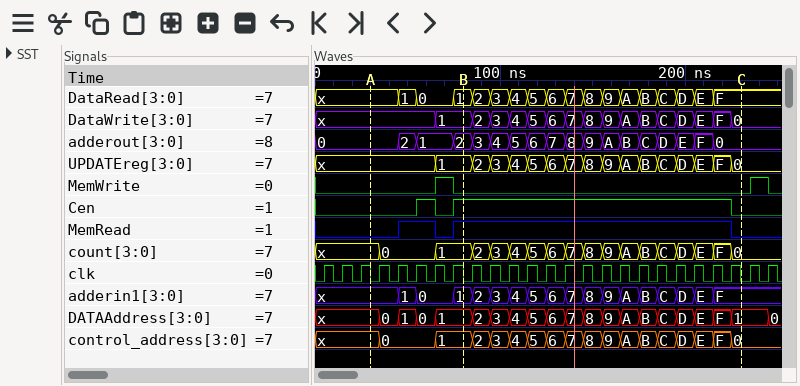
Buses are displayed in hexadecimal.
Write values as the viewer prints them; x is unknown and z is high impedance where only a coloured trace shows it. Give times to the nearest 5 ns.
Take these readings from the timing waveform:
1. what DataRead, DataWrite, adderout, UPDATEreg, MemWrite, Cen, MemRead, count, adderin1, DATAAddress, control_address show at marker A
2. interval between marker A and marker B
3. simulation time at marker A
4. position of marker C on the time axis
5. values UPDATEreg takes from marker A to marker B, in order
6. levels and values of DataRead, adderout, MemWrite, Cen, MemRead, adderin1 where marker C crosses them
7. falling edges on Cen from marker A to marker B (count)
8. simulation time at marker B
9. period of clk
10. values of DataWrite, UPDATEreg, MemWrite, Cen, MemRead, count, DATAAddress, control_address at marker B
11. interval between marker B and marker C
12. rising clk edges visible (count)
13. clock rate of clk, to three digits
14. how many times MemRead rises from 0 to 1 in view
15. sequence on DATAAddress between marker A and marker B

DataRead=x, DataWrite=x, adderout=0, UPDATEreg=x, MemWrite=0, Cen=0, MemRead=0, count=x, adderin1=x, DATAAddress=x, control_address=x
50 ns
30 ns
230 ns
x, 1
DataRead=F, adderout=0, MemWrite=0, Cen=0, MemRead=0, adderin1=F
1
80 ns
10 ns
DataWrite=1, UPDATEreg=1, MemWrite=0, Cen=1, MemRead=1, count=1, DATAAddress=1, control_address=1
150 ns
25
100 MHz
2
x, 0, 1, 0, 1
